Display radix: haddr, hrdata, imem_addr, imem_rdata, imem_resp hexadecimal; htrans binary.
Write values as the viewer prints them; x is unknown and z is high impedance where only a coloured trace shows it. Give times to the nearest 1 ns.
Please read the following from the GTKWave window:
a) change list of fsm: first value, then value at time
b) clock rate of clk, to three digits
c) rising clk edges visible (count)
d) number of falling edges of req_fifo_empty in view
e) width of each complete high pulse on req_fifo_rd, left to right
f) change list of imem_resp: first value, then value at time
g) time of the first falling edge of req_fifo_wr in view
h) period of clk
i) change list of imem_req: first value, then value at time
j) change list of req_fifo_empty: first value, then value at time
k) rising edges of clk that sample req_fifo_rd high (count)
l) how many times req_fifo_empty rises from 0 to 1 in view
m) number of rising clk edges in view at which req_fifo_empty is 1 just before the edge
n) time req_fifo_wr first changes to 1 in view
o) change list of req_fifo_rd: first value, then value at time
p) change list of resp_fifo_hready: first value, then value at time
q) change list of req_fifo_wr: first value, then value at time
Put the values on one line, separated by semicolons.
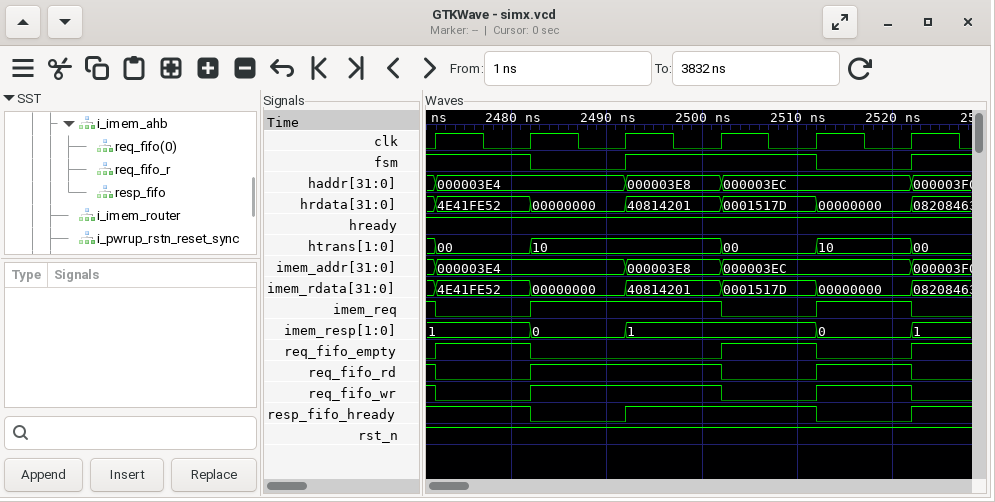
1, 0 at 2482 ns, 1 at 2492 ns, 0 at 2512 ns, 1 at 2522 ns; 100 MHz; 6; 2; 20 ns, 10 ns; 1, 0 at 2482 ns, 1 at 2492 ns, 0 at 2512 ns, 1 at 2522 ns; 2472 ns; 10 ns; 1, 0 at 2472 ns, 1 at 2482 ns, 0 at 2502 ns, 1 at 2512 ns, 0 at 2522 ns; 0, 1 at 2472 ns, 0 at 2482 ns, 1 at 2502 ns, 0 at 2512 ns, 1 at 2522 ns; 4; 3; 2; 2482 ns; 1, 0 at 2472 ns, 1 at 2482 ns, 0 at 2502 ns, 1 at 2512 ns, 0 at 2522 ns; 1, 0 at 2482 ns, 1 at 2492 ns, 0 at 2512 ns, 1 at 2522 ns; 1, 0 at 2472 ns, 1 at 2482 ns, 0 at 2502 ns, 1 at 2512 ns, 0 at 2522 ns
